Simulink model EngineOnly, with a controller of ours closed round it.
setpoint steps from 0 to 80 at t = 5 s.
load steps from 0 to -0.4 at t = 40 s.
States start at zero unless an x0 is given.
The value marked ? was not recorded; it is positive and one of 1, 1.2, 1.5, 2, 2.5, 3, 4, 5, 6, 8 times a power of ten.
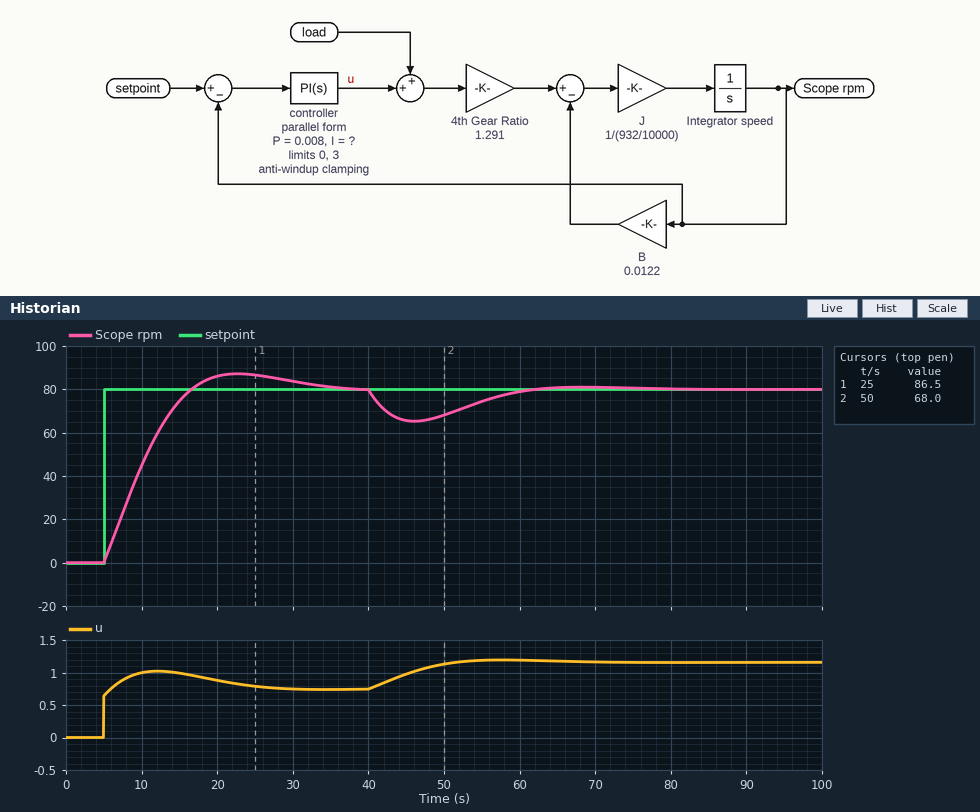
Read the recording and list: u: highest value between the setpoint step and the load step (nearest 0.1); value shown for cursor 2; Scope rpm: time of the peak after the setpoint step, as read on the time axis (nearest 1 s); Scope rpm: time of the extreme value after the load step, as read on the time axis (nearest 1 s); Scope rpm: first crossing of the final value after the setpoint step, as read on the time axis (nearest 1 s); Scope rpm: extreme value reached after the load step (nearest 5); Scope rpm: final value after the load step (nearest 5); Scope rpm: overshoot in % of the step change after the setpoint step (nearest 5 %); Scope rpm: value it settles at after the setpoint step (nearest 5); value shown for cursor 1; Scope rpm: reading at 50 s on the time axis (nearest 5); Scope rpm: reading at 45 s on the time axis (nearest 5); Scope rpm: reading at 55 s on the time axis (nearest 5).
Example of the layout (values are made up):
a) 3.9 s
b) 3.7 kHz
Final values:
a) 1.0
b) 68.0
c) 23 s
d) 46 s
e) 17 s
f) 65
g) 80
h) 10 %
i) 80
j) 86.5
k) 70
l) 65
m) 75
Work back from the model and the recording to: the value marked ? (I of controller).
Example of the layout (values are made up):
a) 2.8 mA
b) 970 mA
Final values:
a) 0.0025
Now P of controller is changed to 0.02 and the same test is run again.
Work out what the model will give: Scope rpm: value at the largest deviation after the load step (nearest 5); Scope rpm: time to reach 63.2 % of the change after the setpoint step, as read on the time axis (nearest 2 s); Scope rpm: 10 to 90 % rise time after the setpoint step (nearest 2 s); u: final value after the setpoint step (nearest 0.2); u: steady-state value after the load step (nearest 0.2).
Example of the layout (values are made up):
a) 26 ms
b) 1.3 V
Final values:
a) 70
b) 8 s
c) 8 s
d) 0.8
e) 1.2
